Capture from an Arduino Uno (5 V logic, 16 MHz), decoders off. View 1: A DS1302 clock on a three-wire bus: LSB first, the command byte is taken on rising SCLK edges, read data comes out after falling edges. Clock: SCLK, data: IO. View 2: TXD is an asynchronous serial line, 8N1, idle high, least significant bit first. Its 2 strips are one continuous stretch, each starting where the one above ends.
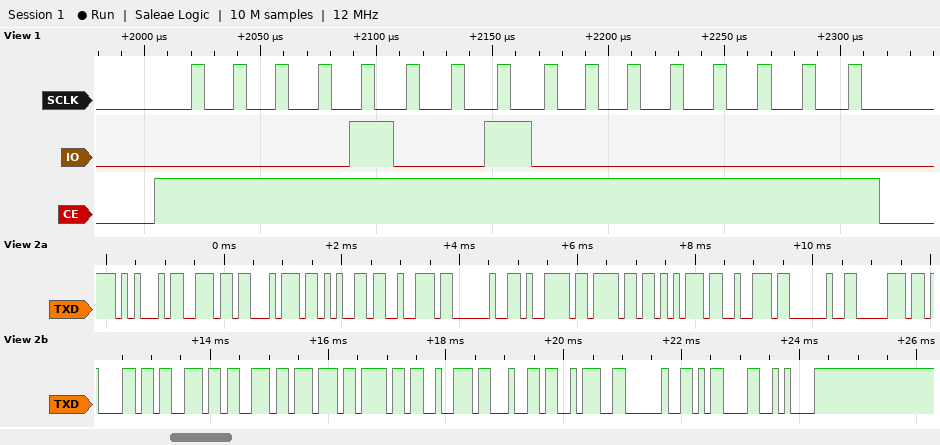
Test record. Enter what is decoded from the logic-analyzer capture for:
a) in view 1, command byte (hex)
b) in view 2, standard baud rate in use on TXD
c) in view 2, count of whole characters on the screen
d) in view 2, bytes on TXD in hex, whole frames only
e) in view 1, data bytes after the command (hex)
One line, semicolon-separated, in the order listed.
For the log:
0x90; 9600 baud; 23; 0x45 0x6E 0x74 0x65 0x72 0x20 0x79 0x6F 0x75 0x72 0x20 0x70 0x61 0x73 0x73 0x77 0x6F 0x72 0x64 0x3A 0x20 0x0D 0x0A; 00
